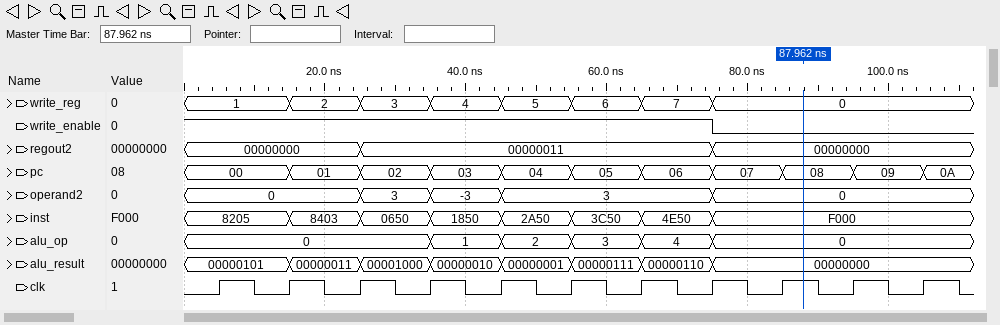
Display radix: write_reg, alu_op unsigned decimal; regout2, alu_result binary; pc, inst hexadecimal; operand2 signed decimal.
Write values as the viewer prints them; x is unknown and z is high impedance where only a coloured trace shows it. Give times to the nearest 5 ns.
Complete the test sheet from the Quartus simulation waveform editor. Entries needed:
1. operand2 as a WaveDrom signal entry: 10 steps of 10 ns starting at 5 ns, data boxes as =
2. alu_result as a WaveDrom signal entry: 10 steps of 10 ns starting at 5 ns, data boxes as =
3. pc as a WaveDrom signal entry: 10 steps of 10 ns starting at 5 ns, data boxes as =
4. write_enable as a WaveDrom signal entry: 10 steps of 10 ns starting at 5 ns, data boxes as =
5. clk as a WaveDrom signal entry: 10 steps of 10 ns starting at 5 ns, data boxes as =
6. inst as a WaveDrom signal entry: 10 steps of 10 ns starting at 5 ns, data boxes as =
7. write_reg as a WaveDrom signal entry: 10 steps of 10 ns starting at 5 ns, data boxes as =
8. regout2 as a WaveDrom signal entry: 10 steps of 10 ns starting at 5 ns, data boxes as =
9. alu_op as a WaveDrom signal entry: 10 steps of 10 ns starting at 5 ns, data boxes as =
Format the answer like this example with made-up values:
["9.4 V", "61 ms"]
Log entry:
["{name: 'operand2', wave: '=.===..=..', data: '0 3 -3 3 0'}", "{name: 'alu_result', wave: '========..', data: '00000101 00000011 00001000 00000010 00000001 00000111 00000110 00000000'}", "{name: 'pc', wave: '==========', data: '00 01 02 03 04 05 06 07 08 09'}", "{name: 'write_enable', wave: '1......0..'}", "{name: 'clk', wave: 'p.........'}", "{name: 'inst', wave: '========..', data: '8205 8403 0650 1850 2A50 3C50 4E50 F000'}", "{name: 'write_reg', wave: '========..', data: '1 2 3 4 5 6 7 0'}", "{name: 'regout2', wave: '=.=....=..', data: '00000000 00000011 00000000'}", "{name: 'alu_op', wave: '=..=====..', data: '0 1 2 3 4 0'}"]
